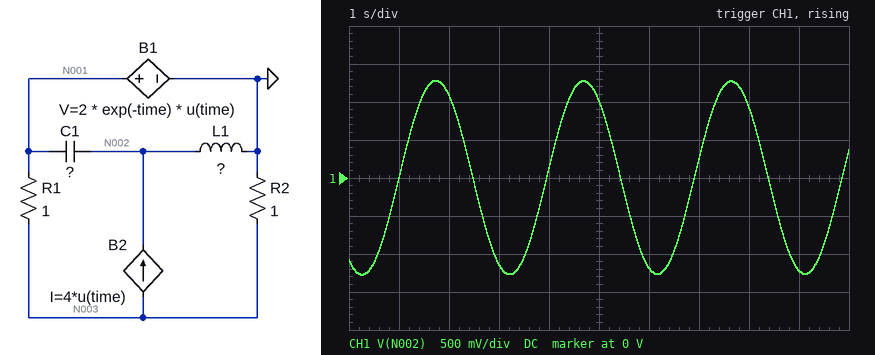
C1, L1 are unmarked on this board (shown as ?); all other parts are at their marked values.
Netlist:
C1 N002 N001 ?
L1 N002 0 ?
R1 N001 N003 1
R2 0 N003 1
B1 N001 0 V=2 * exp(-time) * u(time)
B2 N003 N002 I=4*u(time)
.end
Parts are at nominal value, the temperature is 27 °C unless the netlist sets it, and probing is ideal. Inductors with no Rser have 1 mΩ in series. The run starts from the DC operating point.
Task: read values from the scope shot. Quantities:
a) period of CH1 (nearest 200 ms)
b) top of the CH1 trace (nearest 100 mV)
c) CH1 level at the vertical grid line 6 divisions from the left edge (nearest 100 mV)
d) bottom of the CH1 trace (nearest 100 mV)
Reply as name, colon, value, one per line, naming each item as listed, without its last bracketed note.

period of CH1: 3.0 s
top of the CH1 trace: 1.3 V
CH1 level at the vertical grid line 6 divisions from the left edge: -1.2 V
bottom of the CH1 trace: -1.3 V
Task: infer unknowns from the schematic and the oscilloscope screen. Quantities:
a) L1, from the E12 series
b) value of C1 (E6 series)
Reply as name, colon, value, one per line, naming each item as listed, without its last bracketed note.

L1, from the E12 series: 470 mH
value of C1: 470 mF
